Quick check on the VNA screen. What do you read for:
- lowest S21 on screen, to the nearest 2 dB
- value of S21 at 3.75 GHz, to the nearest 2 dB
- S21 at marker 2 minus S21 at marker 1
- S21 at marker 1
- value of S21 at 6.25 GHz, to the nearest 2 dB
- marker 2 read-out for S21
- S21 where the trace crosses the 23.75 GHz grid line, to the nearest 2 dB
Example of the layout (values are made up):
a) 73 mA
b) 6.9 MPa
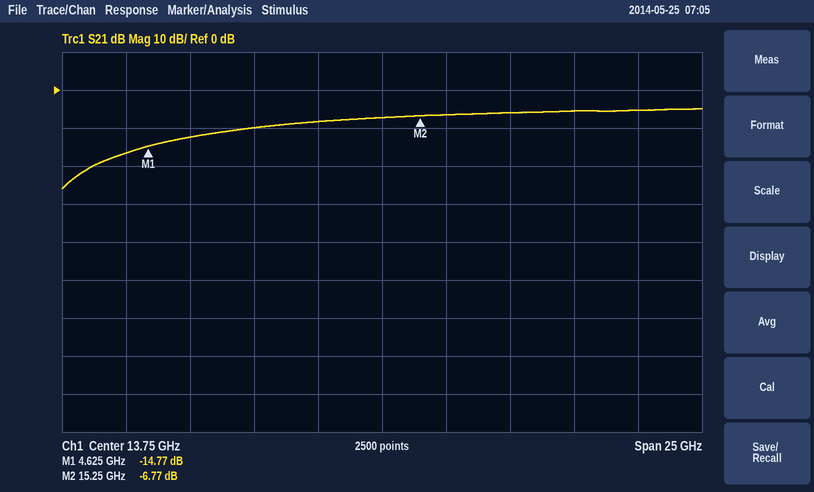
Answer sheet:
a) -26 dB
b) -16 dB
c) 8.00 dB
d) -14.77 dB
e) -12 dB
f) -6.77 dB
g) -6 dB
